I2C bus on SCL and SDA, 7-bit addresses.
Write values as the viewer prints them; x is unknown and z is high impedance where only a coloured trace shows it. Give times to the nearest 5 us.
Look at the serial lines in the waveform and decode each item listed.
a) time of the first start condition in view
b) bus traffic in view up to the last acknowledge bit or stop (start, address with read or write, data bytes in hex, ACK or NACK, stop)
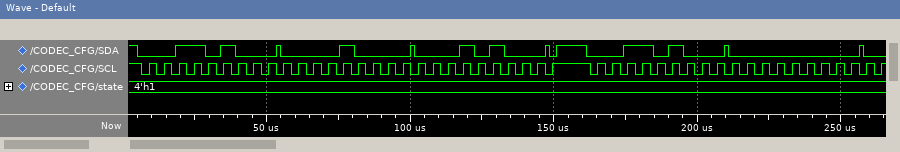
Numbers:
5 us
start, address 1A write ACK, 08 ACK, 14 ACK, stop, start, address 1A write ACK, 00 ACK
